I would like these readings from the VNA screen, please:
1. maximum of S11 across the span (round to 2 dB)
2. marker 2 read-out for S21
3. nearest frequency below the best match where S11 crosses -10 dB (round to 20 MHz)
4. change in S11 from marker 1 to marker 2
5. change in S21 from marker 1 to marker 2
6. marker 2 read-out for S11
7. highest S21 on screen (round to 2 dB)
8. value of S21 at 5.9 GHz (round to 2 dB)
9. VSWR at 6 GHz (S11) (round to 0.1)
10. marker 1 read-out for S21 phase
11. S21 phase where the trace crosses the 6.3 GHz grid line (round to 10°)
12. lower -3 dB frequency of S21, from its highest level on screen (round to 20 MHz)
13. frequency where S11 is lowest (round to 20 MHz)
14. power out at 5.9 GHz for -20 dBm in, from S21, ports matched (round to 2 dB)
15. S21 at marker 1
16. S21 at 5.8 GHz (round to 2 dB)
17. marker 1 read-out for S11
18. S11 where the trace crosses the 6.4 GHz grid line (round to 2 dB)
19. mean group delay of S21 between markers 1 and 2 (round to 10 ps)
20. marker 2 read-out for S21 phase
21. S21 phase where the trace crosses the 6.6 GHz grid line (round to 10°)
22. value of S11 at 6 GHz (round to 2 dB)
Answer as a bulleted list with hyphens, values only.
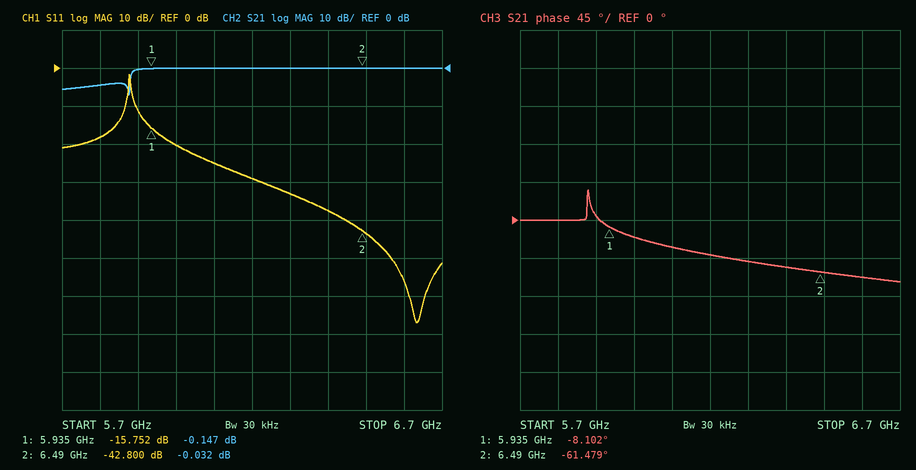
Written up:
- -2 dB
- -0.032 dB
- 5.90 GHz
- -27.048 dB
- 0.115 dB
- -42.800 dB
- 0 dB
- 0 dB
- 1.2
- -8.102°
- -50°
- 5.88 GHz
- 6.64 GHz
- -20 dBm
- -0.147 dB
- -4 dB
- -15.752 dB
- -38 dB
- 270 ps
- -61.479°
- -70°
- -20 dB
